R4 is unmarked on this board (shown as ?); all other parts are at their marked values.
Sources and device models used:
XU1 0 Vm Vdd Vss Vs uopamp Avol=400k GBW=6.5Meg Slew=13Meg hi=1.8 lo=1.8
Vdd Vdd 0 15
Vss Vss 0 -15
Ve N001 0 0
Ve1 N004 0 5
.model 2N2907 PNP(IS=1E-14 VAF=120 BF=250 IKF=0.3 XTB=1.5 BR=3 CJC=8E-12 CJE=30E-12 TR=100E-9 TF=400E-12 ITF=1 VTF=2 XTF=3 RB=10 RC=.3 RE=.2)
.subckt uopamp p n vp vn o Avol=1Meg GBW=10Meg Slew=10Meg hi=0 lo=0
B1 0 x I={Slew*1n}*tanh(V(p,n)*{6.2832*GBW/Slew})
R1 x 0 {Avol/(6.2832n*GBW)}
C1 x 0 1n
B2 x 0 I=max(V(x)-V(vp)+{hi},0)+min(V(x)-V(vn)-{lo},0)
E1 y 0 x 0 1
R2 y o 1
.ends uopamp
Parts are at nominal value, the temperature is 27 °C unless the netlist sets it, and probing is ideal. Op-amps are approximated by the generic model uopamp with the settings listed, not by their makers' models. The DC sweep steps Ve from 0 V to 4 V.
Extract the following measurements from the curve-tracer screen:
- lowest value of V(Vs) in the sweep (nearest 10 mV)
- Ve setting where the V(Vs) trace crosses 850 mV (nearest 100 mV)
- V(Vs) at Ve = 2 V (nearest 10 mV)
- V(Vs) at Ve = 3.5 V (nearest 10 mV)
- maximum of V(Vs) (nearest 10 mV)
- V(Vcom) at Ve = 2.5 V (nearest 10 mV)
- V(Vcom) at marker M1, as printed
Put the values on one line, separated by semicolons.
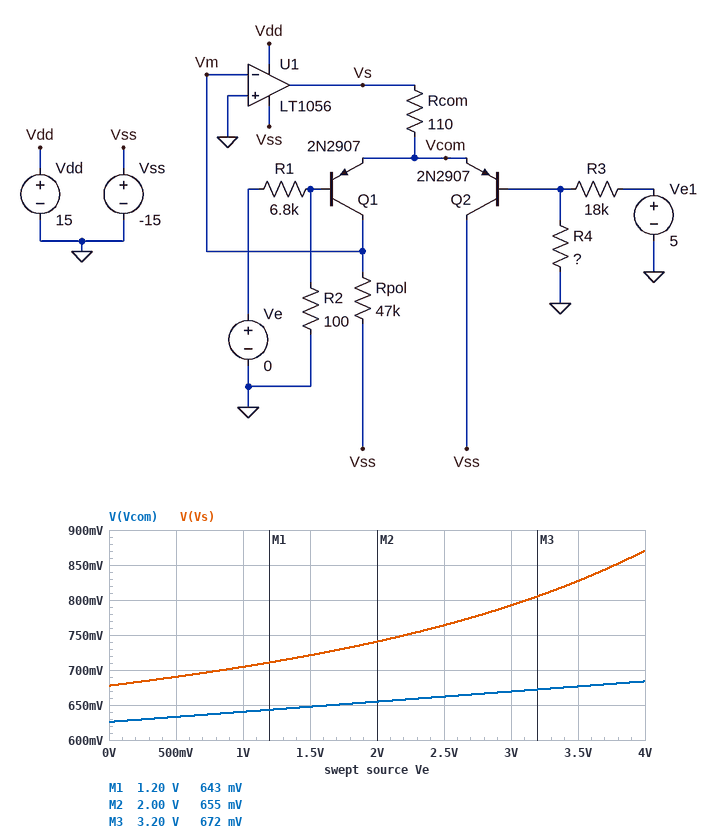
680 mV; 3.8 V; 740 mV; 830 mV; 870 mV; 660 mV; 643 mV
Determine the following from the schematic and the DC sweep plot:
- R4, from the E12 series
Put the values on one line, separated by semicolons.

82 Ω
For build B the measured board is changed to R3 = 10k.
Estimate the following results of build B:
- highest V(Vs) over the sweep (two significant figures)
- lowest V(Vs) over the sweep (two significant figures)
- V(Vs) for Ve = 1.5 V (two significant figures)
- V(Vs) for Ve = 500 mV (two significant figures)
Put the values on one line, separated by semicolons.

800 mV; 670 mV; 700 mV; 680 mV
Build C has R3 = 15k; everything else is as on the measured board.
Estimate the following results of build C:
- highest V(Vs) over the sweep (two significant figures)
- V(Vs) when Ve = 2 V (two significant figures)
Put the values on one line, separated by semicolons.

850 mV; 730 mV
